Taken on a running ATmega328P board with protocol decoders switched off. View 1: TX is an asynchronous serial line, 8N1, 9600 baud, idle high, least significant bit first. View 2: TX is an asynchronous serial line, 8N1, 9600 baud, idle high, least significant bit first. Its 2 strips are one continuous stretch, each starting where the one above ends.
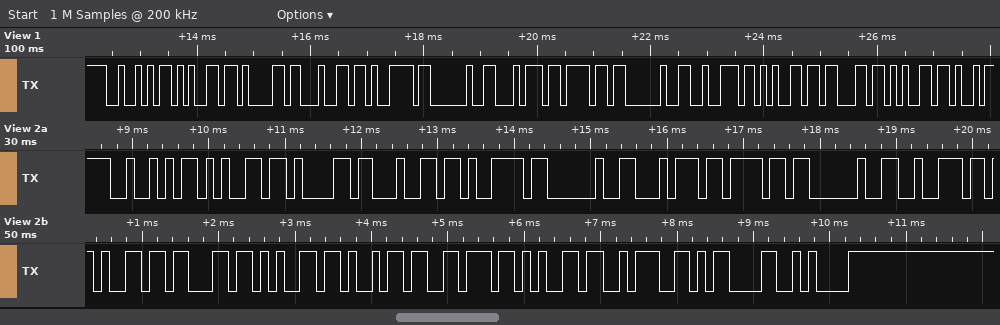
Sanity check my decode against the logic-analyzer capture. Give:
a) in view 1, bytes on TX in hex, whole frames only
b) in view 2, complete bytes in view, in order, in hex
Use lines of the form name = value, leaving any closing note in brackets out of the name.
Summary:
in view 1, bytes on TX in hex, whole frames only = 52 65 61 64 79 20 74 6F 20 72 65 63 65
in view 2, complete bytes in view, in order, in hex = 0x52 0x65 0x61 0x64 0x79 0x20 0x74 0x6F 0x20 0x72 0x65 0x63 0x65 0x69 0x76 0x65 0x3A 0x0D 0x0A
